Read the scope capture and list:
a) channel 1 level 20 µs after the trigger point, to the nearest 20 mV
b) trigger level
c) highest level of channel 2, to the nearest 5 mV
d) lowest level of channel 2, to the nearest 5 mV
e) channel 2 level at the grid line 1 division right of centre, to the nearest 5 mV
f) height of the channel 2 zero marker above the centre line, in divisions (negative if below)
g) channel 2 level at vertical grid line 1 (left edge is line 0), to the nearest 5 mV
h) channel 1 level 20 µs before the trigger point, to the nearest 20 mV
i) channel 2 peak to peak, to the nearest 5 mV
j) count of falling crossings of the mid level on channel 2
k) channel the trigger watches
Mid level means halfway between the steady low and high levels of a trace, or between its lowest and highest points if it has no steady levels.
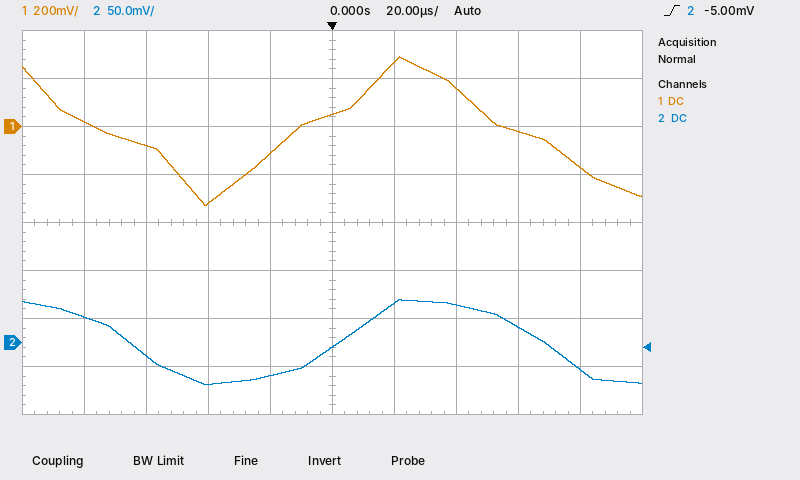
260 mV
-5.00 mV
45 mV
-45 mV
40 mV
-2.5 div
25 mV
-120 mV
90 mV
2
channel 2
